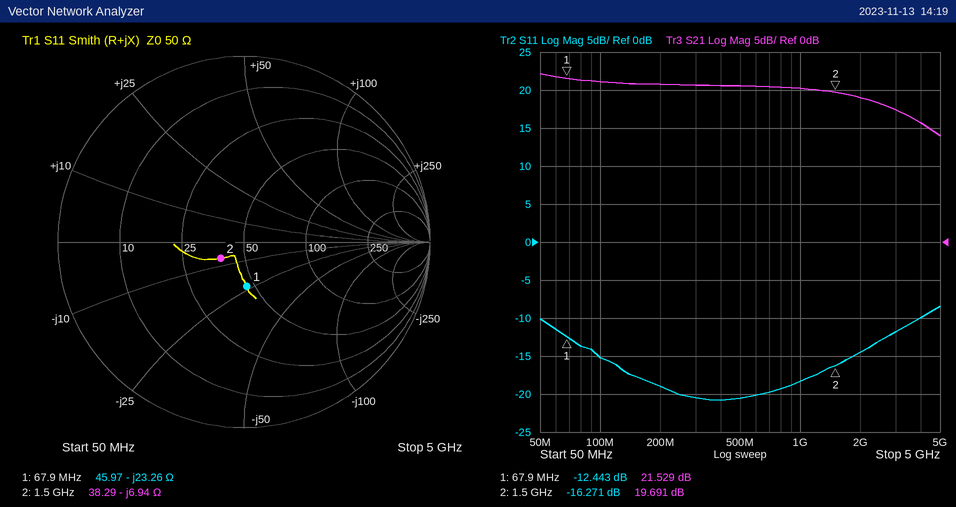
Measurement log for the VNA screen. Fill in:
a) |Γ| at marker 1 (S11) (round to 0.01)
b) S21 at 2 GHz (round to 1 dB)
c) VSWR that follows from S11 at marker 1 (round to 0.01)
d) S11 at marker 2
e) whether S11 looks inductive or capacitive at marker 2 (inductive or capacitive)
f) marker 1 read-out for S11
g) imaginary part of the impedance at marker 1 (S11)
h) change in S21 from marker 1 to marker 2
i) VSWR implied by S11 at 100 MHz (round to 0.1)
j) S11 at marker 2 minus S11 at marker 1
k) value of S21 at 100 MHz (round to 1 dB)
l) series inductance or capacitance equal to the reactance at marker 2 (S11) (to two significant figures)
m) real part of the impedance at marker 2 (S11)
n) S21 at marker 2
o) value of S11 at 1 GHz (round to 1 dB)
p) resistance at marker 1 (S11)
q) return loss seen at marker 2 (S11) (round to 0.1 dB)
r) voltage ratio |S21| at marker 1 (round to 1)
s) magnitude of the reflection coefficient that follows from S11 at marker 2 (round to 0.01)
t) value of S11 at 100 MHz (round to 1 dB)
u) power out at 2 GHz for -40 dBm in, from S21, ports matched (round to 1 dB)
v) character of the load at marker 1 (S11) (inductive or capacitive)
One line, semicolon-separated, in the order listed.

0.24; 19 dB; 1.63; -16.271 dB; capacitive; -12.443 dB; -23.26 Ω; -1.838 dB; 1.4; -3.828 dB; 21 dB; 15 pF; 38.29 Ω; 19.691 dB; -18 dB; 45.97 Ω; 16.3 dB; 12; 0.15; -15 dB; -21 dBm; capacitive
